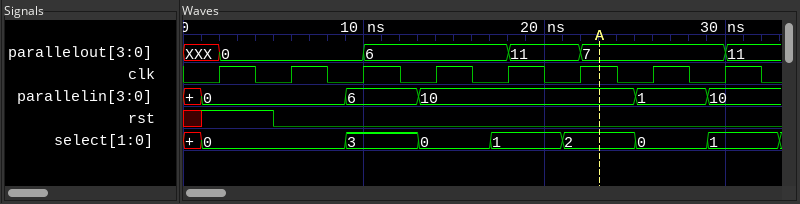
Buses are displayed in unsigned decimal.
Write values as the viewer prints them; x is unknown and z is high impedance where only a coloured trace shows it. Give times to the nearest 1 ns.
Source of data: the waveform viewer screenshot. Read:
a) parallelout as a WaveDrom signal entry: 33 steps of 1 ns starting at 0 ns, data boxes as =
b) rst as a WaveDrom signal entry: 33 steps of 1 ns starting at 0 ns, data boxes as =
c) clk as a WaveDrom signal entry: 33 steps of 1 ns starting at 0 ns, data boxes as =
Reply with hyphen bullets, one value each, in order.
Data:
- {name: 'parallelout', wave: 'x.=.......=.......=...=.......=..', data: '0 6 11 7 11'}
- {name: 'rst', wave: 'x1...0...........................'}
- {name: 'clk', wave: '0.1.0.1.0.1.0.1.0.1.0.1.0.1.0.1.0'}
